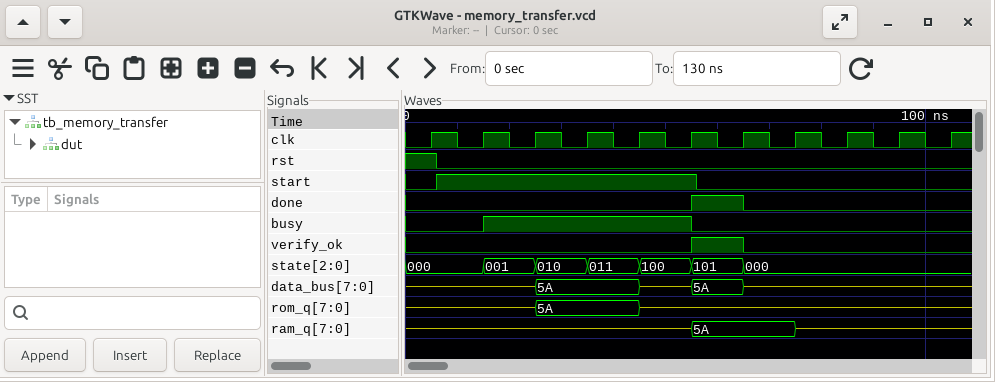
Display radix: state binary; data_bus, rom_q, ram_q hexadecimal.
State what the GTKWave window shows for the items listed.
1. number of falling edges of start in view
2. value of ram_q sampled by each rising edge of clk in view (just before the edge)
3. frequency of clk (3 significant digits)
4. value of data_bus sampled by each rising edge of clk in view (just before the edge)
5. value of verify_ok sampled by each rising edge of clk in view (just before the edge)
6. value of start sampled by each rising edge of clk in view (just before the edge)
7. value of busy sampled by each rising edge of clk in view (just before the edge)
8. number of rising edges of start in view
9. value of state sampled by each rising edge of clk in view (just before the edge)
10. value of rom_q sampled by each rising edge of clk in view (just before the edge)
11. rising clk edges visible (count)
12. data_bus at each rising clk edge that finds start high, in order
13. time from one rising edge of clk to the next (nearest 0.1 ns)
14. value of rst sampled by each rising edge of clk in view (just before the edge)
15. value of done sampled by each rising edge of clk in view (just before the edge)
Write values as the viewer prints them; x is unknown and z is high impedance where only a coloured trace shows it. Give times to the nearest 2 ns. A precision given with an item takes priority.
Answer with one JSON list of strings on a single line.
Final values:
["1", "z, z, z, z, z, z, 5A, 5A, z, z, z", "100 MHz", "z, z, z, 5A, 5A, z, 5A, z, z, z, z", "0 0 0 0 0 0 1 0 0 0 0", "0 1 1 1 1 1 0 0 0 0 0", "0 0 1 1 1 1 0 0 0 0 0", "1", "000, 000, 001, 010, 011, 100, 101, 000, 000, 000, 000", "z, z, z, 5A, 5A, z, z, z, z, z, z", "11", "z, z, 5A, 5A, z", "10 ns", "1 0 0 0 0 0 0 0 0 0 0", "0 0 0 0 0 0 1 0 0 0 0"]
